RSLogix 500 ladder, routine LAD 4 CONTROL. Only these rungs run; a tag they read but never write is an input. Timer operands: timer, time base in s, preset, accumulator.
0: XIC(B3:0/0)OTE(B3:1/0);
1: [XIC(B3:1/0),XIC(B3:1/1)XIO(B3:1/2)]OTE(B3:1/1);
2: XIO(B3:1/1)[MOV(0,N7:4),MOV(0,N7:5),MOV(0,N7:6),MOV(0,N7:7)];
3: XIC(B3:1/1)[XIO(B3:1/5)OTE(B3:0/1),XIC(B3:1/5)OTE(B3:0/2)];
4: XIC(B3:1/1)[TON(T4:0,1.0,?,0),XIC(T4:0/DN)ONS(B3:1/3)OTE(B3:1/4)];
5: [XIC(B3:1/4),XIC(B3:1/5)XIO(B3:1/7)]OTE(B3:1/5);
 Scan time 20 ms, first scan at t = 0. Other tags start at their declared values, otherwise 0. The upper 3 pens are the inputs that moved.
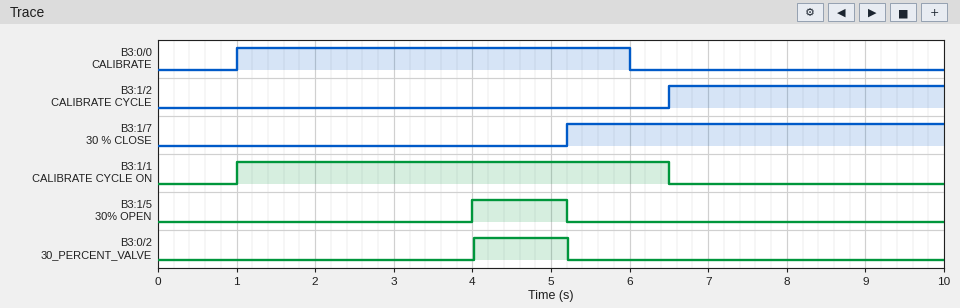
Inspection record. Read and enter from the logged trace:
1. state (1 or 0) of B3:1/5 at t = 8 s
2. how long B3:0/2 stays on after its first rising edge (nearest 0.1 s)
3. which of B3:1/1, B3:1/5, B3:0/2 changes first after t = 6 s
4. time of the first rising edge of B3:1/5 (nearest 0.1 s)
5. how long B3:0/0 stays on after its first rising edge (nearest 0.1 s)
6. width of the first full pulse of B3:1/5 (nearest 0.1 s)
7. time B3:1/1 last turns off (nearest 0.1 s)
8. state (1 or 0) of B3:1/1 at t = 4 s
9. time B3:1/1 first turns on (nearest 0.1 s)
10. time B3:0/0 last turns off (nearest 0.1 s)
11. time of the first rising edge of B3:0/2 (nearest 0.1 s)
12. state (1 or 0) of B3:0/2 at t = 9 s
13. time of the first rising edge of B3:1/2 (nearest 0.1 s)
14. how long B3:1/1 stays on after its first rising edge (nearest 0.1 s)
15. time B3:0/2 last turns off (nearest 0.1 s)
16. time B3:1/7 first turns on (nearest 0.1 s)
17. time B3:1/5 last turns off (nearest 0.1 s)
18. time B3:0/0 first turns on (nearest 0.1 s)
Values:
0
1.2 s
B3:1/1
4.0 s
5.0 s
1.2 s
6.5 s
1
1.0 s
6.0 s
4.0 s
0
6.5 s
5.5 s
5.2 s
5.2 s
5.2 s
1.0 s
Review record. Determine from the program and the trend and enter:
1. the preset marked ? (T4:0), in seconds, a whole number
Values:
3 s
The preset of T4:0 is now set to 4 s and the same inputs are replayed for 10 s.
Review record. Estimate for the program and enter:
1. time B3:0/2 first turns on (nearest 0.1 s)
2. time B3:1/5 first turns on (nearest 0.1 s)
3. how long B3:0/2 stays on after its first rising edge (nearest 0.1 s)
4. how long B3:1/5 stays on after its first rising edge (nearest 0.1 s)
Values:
5.0 s
5.0 s
0.2 s
0.2 s
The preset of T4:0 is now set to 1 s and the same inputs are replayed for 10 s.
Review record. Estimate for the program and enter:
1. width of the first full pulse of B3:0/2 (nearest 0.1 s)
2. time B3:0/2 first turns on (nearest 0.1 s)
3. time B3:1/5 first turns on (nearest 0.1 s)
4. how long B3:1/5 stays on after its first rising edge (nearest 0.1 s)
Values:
3.2 s
2.0 s
2.0 s
3.2 s
